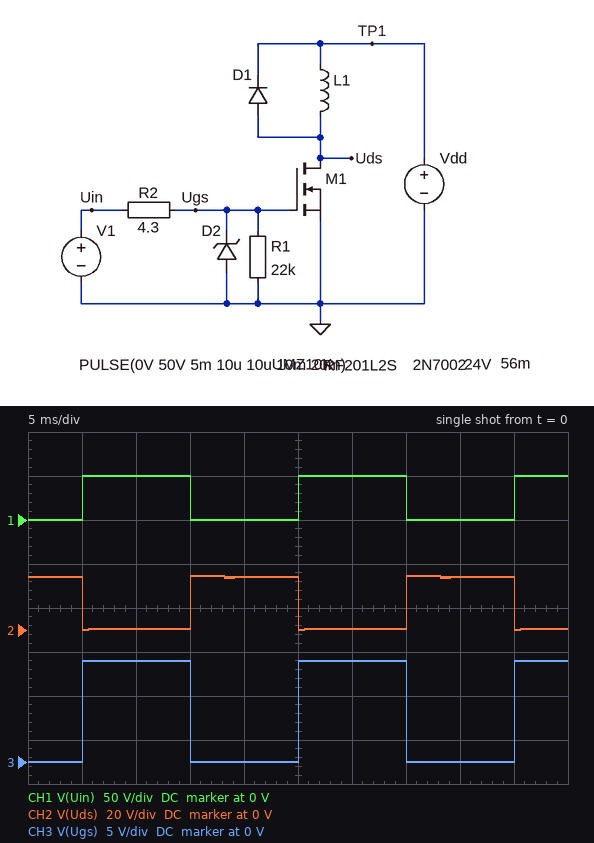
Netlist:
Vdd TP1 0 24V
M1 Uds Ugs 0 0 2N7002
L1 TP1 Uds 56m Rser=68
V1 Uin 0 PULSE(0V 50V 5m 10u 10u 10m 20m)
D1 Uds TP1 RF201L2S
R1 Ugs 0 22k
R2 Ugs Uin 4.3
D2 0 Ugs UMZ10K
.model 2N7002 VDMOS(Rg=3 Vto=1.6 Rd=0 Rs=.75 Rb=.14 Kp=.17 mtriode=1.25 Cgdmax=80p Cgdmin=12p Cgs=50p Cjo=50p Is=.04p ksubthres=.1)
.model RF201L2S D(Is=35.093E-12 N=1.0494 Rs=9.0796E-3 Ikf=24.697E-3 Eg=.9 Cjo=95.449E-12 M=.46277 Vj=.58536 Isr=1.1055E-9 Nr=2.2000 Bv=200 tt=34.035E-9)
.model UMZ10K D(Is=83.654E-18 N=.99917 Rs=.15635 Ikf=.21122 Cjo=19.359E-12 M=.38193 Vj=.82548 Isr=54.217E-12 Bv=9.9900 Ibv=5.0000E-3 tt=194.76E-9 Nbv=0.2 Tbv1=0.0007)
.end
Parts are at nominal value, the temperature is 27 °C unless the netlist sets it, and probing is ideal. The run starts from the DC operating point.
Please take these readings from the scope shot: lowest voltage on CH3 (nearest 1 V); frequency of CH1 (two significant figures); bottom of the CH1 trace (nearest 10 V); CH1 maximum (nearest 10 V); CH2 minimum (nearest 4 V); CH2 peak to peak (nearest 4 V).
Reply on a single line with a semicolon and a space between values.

0 V; 50 Hz; 0 V; 50 V; 0 V; 24 V
